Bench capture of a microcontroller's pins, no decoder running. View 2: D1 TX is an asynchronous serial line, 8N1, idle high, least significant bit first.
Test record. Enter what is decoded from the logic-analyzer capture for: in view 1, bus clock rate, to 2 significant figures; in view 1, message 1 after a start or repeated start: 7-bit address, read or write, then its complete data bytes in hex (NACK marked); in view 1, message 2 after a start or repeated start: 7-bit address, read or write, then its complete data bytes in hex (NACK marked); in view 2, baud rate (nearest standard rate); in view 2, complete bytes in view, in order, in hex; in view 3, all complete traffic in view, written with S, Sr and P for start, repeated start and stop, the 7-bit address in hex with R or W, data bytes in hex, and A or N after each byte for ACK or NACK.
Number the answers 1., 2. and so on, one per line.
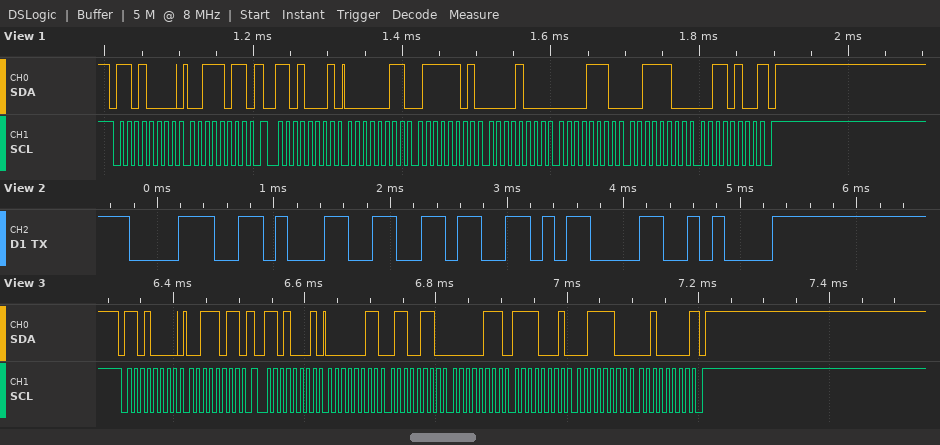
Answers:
1. 100 kHz
2. 0x68 write: 3B
3. 0x68 read: 03 7D 08 0E 3C 34 NACK
4. 9600 baud
5. 38 31 36 0D 0A
6. S 68W A 3B A Sr 68R A 03 A 66 A 07 A F1 A 3C A 20 N P
